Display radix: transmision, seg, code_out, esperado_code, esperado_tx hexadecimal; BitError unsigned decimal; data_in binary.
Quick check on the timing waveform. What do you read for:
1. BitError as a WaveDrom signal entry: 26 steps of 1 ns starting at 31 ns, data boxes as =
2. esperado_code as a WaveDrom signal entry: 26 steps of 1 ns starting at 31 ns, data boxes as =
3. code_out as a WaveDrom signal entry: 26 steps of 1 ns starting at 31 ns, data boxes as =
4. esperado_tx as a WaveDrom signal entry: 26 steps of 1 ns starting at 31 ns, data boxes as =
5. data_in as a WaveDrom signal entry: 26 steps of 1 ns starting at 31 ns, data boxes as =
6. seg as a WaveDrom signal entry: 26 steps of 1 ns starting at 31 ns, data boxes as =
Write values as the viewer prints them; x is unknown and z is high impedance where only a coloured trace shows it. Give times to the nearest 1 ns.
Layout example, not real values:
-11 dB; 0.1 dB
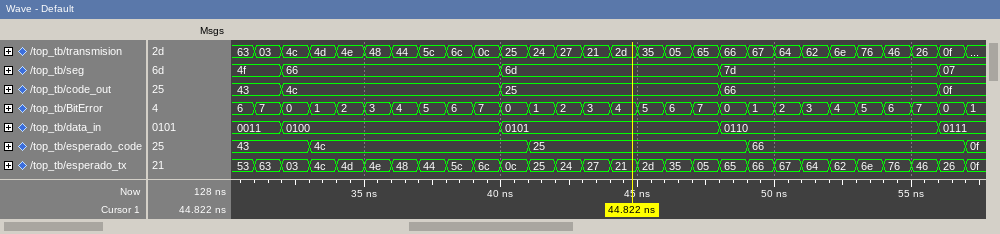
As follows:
{name: 'BitError', wave: '==========================', data: '7 0 1 2 3 4 5 6 7 0 1 2 3 4 5 6 7 0 1 2 3 4 5 6 7 0'}; {name: 'esperado_code', wave: '=.=.......=.......=.......', data: '43 4c 25 66'}; {name: 'code_out', wave: '==.......=.......=.......=', data: '43 4c 25 66 0f'}; {name: 'esperado_tx', wave: '==========================', data: '63 03 4c 4d 4e 48 44 5c 6c 0c 25 24 27 21 2d 35 05 65 66 67 64 62 6e 76 46 26'}; {name: 'data_in', wave: '==.......=.......=.......=', data: '0011 0100 0101 0110 0111'}; {name: 'seg', wave: '==.......=.......=.......=', data: '4f 66 6d 7d 07'}
